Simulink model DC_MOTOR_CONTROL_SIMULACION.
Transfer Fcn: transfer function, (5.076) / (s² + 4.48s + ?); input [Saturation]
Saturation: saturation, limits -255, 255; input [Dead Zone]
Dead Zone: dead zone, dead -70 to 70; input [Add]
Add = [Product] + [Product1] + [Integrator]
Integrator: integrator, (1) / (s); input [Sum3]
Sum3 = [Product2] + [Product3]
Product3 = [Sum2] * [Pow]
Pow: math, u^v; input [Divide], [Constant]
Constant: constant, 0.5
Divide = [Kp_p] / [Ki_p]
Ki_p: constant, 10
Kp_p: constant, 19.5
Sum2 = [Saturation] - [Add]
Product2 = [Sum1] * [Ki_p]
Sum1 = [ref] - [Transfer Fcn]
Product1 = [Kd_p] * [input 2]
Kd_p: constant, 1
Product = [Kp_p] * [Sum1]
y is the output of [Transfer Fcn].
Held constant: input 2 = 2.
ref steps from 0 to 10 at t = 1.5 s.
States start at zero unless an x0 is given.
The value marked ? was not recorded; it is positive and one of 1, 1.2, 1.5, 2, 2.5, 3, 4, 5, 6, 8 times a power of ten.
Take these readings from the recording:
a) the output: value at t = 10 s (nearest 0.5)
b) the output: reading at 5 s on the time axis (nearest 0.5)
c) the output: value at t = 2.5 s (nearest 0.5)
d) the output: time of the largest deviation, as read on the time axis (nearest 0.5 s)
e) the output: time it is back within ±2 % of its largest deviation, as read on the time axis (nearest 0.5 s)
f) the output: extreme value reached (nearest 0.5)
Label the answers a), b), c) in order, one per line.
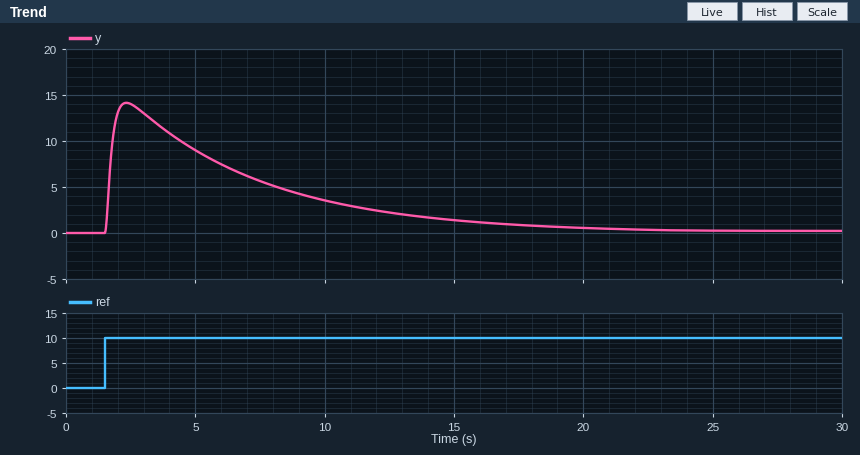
a) 3.5
b) 9.0
c) 14.0
d) 2.5 s
e) 20.5 s
f) 14.0
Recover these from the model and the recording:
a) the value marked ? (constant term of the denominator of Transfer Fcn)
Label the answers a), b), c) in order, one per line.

a) 0.8
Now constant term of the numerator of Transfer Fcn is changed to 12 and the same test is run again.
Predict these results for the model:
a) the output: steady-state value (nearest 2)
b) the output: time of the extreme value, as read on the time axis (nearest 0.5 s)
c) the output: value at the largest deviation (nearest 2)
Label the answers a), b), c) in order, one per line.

a) 0
b) 2.0 s
c) 16
